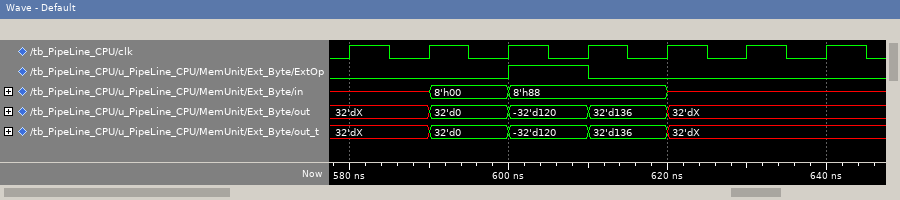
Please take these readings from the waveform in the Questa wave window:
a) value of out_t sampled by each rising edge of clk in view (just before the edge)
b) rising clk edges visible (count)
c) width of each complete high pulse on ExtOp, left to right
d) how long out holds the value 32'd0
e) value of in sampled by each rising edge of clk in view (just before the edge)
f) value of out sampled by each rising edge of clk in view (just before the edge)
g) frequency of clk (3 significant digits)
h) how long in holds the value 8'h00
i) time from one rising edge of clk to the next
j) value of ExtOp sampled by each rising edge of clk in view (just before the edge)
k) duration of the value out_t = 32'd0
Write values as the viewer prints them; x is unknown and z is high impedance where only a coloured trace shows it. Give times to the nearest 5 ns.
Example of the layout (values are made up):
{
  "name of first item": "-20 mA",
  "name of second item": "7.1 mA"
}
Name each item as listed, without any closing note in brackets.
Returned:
{
  "value of out_t sampled by each rising edge of clk in view": "32'dX, 32'dX, 32'd0, -32'd120, 32'd136, 32'dX, 32'dX",
  "rising clk edges visible": "7",
  "width of each complete high pulse on ExtOp, left to right": "10 ns",
  "how long out holds the value 32'd0": "10 ns",
  "value of in sampled by each rising edge of clk in view": "x, x, 8'h00, 8'h88, 8'h88, x, x",
  "value of out sampled by each rising edge of clk in view": "32'dX, 32'dX, 32'd0, -32'd120, 32'd136, 32'dX, 32'dX",
  "frequency of clk": "100 MHz",
  "how long in holds the value 8'h00": "10 ns",
  "time from one rising edge of clk to the next": "10 ns",
  "value of ExtOp sampled by each rising edge of clk in view": "0 0 0 1 0 0 0",
  "duration of the value out_t = 32'd0": "10 ns"
}
